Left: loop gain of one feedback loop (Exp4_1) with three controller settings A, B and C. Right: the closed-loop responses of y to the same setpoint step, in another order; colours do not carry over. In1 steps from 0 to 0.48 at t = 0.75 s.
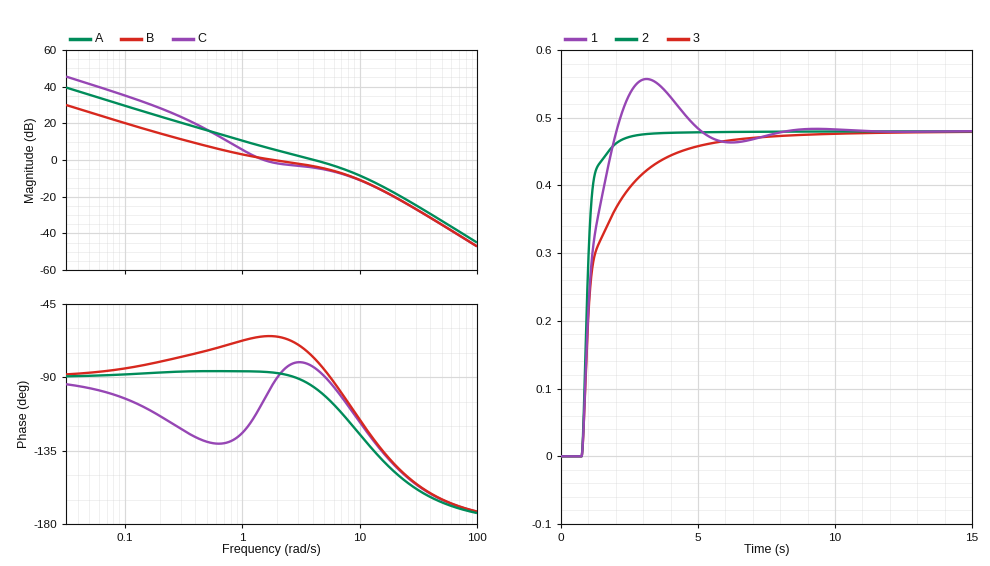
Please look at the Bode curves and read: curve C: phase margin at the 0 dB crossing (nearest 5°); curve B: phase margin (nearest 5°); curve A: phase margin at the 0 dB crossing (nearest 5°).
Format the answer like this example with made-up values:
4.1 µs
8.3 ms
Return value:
75°
115°
85°
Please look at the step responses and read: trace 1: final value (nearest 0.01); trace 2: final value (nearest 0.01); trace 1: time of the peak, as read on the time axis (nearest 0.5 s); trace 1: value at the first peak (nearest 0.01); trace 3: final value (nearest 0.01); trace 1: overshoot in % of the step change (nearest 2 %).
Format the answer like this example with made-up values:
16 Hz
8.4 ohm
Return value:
0.48
0.48
3.0 s
0.56
0.48
16 %
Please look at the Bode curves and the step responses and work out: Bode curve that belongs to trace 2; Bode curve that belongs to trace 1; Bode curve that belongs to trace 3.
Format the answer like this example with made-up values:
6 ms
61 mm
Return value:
A
C
B
